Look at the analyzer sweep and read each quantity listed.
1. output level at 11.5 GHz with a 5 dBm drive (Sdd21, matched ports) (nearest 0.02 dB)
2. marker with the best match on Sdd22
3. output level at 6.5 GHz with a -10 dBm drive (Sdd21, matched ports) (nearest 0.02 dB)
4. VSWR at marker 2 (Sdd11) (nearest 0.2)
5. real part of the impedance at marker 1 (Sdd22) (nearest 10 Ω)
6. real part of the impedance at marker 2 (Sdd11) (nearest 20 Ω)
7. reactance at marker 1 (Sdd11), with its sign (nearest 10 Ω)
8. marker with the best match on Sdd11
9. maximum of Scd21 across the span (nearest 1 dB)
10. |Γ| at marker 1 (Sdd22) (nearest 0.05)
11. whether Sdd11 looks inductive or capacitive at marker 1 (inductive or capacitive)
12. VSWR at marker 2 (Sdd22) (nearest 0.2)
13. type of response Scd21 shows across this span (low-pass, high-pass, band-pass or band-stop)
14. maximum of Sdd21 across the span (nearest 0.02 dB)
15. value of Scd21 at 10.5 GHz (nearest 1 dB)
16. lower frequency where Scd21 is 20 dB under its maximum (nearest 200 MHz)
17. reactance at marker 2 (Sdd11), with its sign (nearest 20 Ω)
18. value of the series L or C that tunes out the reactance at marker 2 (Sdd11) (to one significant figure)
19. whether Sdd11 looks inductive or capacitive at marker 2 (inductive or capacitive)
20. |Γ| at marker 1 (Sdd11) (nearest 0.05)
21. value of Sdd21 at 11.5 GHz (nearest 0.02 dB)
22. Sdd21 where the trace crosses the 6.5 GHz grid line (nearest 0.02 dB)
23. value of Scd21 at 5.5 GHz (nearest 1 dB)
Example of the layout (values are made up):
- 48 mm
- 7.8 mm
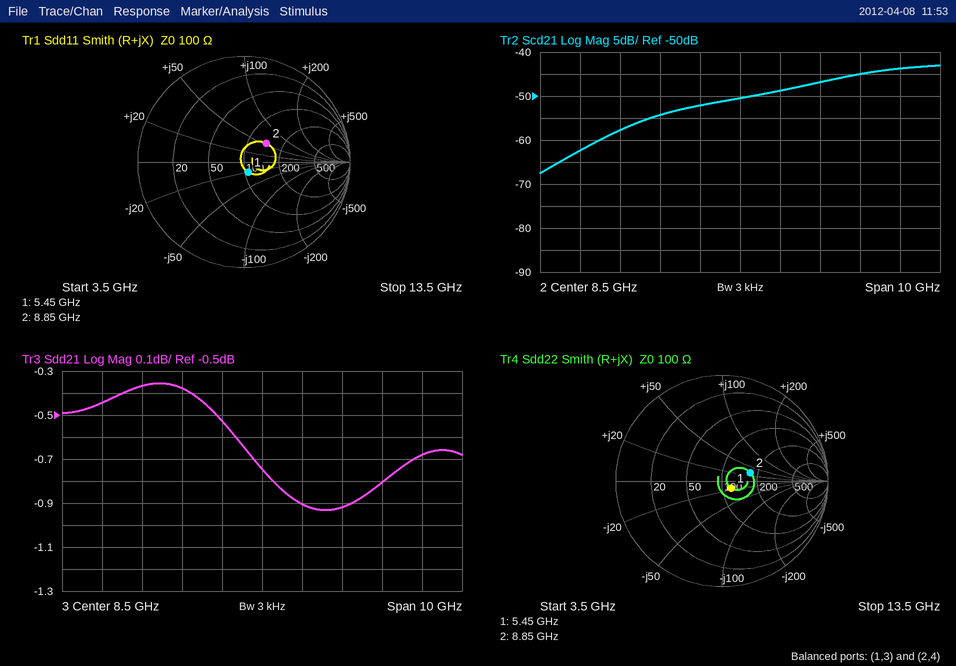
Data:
- 4.20 dBm
- marker 1
- -10.38 dBm
- 1.8
- 120 Ω
- 140 Ω
- -20 Ω
- marker 1
- -43 dB
- 0.10
- capacitive
- 1.8
- high-pass
- -0.36 dB
- -47 dB
- 4.4 GHz
- +60 Ω
- 300 fF
- inductive
- 0.10
- -0.80 dB
- -0.38 dB
- -58 dB
